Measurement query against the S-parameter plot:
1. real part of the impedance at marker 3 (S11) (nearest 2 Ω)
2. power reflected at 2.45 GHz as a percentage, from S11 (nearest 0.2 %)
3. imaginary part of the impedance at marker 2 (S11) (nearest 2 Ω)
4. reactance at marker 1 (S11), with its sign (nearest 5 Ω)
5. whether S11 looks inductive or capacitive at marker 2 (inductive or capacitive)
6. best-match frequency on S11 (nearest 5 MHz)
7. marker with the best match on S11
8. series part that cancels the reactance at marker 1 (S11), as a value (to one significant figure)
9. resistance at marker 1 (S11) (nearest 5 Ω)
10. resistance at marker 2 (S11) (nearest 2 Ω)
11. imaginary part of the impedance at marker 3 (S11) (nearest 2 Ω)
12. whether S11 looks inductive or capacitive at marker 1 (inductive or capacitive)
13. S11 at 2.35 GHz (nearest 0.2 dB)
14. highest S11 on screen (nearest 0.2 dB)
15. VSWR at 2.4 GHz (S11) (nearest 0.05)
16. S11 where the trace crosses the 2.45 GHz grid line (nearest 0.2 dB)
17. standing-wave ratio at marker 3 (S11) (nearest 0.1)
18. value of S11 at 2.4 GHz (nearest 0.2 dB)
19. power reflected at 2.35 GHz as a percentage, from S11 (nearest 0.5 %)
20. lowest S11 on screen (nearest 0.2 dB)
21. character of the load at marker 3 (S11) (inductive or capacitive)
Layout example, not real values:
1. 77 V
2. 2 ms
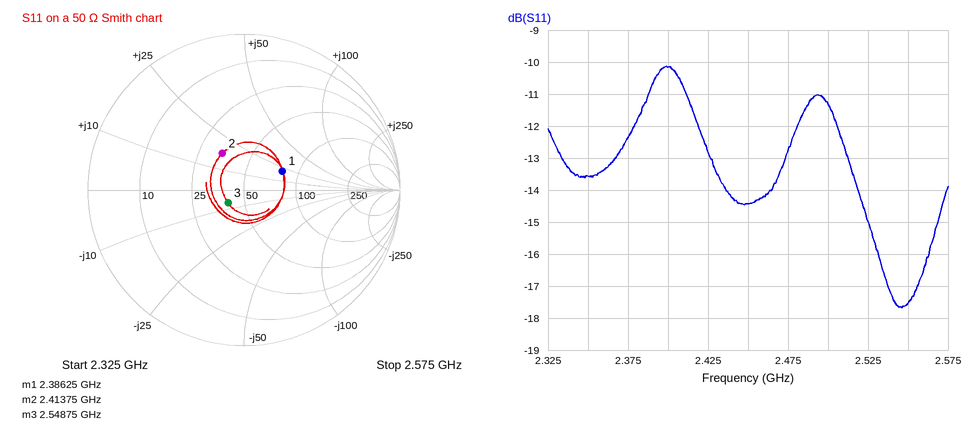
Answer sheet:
1. 40 Ω
2. 3.6 %
3. +18 Ω
4. +20 Ω
5. inductive
6. 2.545 GHz
7. marker 3
8. 3 pF
9. 80 Ω
10. 34 Ω
11. -6 Ω
12. inductive
13. -13.6 dB
14. -10.2 dB
15. 1.90
16. -14.4 dB
17. 1.3
18. -10.2 dB
19. 4.5 %
20. -17.6 dB
21. capacitive
